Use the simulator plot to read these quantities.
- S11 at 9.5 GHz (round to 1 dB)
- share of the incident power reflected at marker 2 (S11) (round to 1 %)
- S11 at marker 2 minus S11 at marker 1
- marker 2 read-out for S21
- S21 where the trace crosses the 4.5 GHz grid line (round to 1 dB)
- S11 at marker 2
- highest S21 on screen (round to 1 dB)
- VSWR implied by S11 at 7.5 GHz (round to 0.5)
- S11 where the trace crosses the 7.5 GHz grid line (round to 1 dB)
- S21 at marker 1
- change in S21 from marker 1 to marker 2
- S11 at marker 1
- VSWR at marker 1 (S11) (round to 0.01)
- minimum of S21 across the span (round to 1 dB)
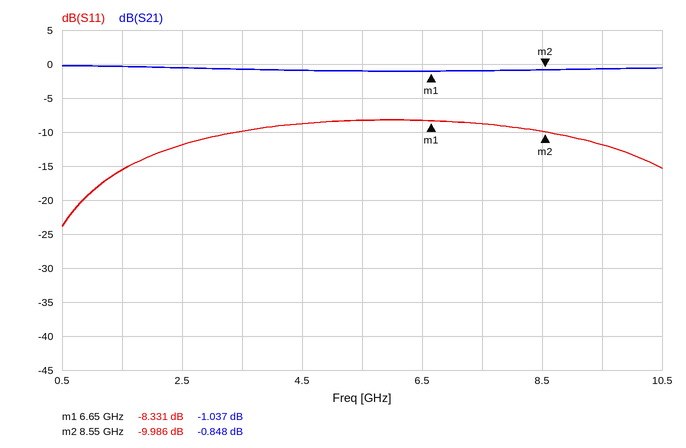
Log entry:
-12 dB
10 %
-1.655 dB
-0.848 dB
-1 dB
-9.986 dB
0 dB
2.0
-9 dB
-1.037 dB
0.189 dB
-8.331 dB
2.24
-1 dB
